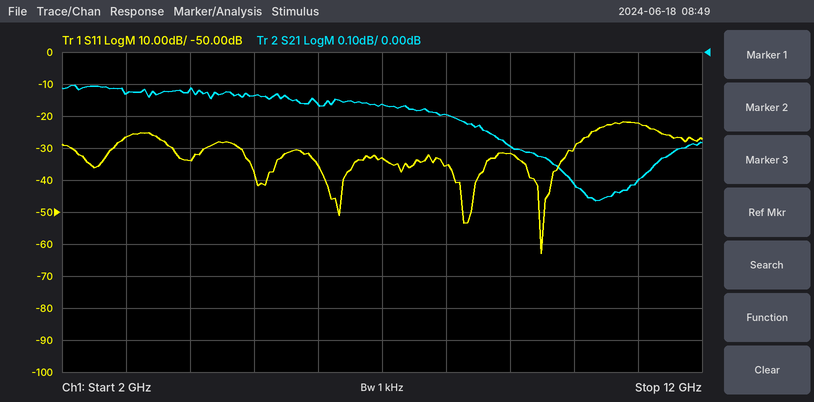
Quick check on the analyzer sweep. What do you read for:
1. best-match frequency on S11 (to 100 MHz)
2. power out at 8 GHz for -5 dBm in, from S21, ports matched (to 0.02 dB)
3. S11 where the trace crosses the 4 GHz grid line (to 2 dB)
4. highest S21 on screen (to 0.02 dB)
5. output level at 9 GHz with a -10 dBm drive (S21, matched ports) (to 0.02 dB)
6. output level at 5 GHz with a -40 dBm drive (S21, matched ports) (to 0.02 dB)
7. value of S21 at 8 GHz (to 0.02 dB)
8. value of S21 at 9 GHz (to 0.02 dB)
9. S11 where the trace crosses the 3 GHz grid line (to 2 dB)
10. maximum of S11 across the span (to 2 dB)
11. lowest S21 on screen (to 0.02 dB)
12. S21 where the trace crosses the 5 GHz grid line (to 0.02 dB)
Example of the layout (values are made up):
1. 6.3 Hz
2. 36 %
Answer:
1. 9.5 GHz
2. -5.20 dBm
3. -34 dB
4. -0.10 dB
5. -10.30 dBm
6. -40.14 dBm
7. -0.20 dB
8. -0.30 dB
9. -26 dB
10. -22 dB
11. -0.46 dB
12. -0.14 dB
